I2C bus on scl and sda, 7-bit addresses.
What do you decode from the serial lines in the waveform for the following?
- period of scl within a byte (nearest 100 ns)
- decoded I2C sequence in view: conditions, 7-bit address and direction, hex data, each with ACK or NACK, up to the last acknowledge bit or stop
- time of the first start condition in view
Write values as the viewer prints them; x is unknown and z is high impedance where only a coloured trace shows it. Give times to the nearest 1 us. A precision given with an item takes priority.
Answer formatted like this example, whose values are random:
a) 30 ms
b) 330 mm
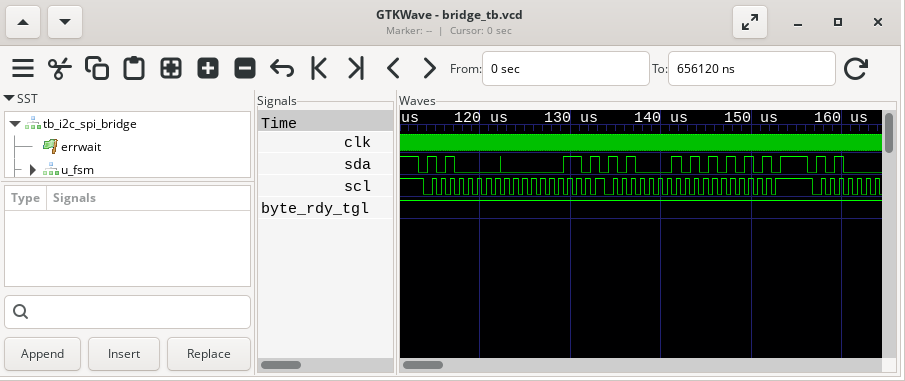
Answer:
a) 1000 ns
b) start, address 50 write ACK, 03 ACK, repeated start, address 50 read ACK, AA NACK, stop
c) 113 us
